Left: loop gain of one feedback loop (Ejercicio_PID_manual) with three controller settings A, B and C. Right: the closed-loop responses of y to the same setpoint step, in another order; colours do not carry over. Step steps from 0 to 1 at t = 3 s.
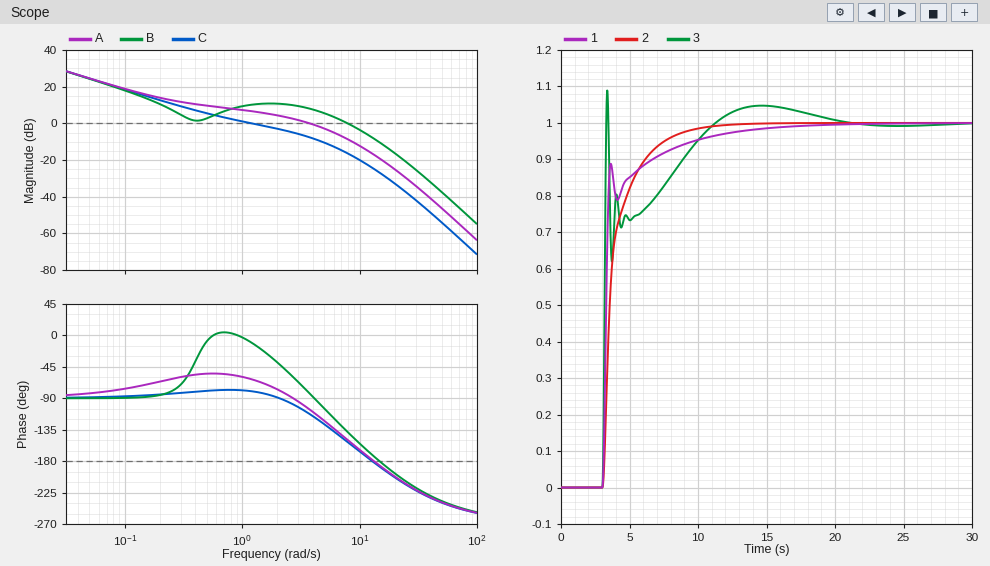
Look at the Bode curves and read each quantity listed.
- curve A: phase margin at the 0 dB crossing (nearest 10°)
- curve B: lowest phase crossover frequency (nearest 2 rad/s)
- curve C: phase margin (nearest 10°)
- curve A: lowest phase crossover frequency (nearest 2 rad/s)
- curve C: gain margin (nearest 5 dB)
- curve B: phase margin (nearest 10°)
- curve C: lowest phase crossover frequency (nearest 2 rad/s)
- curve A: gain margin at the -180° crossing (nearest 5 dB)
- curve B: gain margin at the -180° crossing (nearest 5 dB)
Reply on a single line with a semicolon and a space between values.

70°; 14 rad/s; 100°; 14 rad/s; 25 dB; 40°; 12 rad/s; 15 dB; 10 dB
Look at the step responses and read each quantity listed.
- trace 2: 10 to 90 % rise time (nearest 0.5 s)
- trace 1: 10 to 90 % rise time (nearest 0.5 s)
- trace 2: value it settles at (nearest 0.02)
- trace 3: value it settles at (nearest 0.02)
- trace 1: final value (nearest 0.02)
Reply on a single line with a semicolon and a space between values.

3.0 s; 3.5 s; 1.00; 1.00; 1.00
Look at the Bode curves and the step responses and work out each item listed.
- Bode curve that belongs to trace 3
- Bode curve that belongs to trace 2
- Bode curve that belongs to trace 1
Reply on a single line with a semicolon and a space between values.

B; C; A
